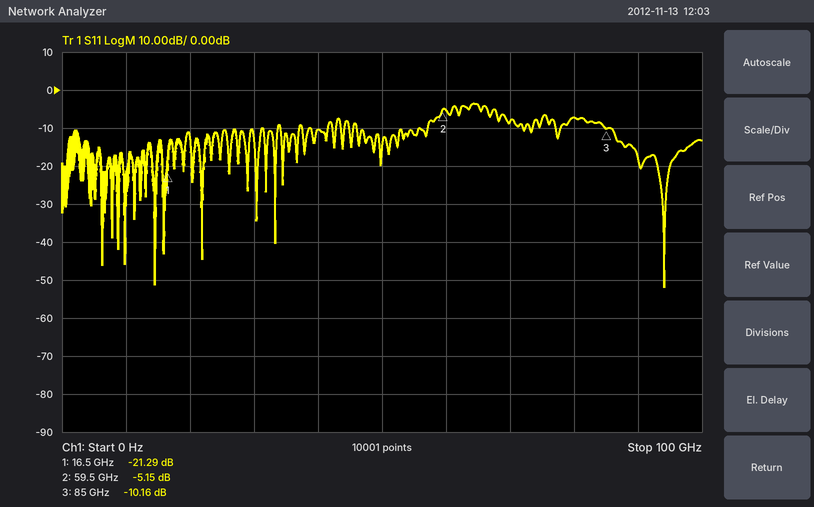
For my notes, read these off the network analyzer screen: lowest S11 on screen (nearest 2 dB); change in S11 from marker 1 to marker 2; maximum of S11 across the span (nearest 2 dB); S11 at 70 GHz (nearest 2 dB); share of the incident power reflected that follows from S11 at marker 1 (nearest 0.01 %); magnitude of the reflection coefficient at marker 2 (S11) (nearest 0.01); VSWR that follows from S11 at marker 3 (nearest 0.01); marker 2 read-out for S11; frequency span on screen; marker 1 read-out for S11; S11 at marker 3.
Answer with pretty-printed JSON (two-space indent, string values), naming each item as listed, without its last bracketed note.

{
  "lowest S11 on screen": "-52 dB",
  "change in S11 from marker 1 to marker 2": "16.14 dB",
  "maximum of S11 across the span": "-4 dB",
  "S11 at 70 GHz": "-8 dB",
  "share of the incident power reflected that follows from S11 at marker 1": "0.74 %",
  "magnitude of the reflection coefficient at marker 2 (S11)": "0.55",
  "VSWR that follows from S11 at marker 3": "1.90",
  "marker 2 read-out for S11": "-5.15 dB",
  "frequency span on screen": "100 GHz",
  "marker 1 read-out for S11": "-21.29 dB",
  "S11 at marker 3": "-10.16 dB"
}
